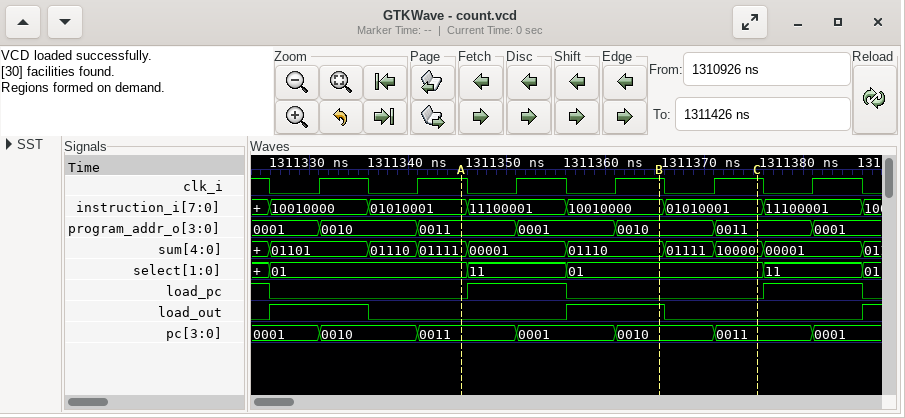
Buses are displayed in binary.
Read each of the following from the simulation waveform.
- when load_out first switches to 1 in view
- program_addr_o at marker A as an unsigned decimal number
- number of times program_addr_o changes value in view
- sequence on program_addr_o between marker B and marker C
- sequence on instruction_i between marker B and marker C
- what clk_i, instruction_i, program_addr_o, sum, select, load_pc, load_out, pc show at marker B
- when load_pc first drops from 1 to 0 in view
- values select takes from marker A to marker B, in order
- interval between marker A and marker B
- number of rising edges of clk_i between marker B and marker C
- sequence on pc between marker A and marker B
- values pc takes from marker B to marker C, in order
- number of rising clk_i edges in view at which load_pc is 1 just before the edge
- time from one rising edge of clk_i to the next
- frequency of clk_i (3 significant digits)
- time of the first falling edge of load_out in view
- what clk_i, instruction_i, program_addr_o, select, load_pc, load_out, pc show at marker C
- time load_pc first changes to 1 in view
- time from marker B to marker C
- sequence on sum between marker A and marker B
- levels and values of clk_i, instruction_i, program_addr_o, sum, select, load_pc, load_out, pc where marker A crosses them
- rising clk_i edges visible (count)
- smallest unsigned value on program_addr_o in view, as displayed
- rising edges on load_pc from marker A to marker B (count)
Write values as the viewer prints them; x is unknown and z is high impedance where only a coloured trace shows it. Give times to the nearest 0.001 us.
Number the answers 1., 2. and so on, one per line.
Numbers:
1. 1311.326 us
2. 3
3. 6
4. 0010, 0011
5. 10010000, 01010001
6. clk_i=1, instruction_i=10010000, program_addr_o=0010, sum=01110, select=01, load_pc=0, load_out=1, pc=0010
7. 1311.326 us
8. 01, 11, 01
9. 0.02 us
10. 1
11. 0011, 0001, 0010
12. 0010, 0011
13. 2
14. 0.01 us
15. 100 MHz
16. 1311.336 us
17. clk_i=1, instruction_i=01010001, program_addr_o=0011, select=01, load_pc=0, load_out=0, pc=0011
18. 1311.346 us
19. 0.01 us
20. 01111, 00001, 01110
21. clk_i=1, instruction_i=01010001, program_addr_o=0011, sum=01111, select=01, load_pc=0, load_out=0, pc=0011
22. 6
23. 0001
24. 1
